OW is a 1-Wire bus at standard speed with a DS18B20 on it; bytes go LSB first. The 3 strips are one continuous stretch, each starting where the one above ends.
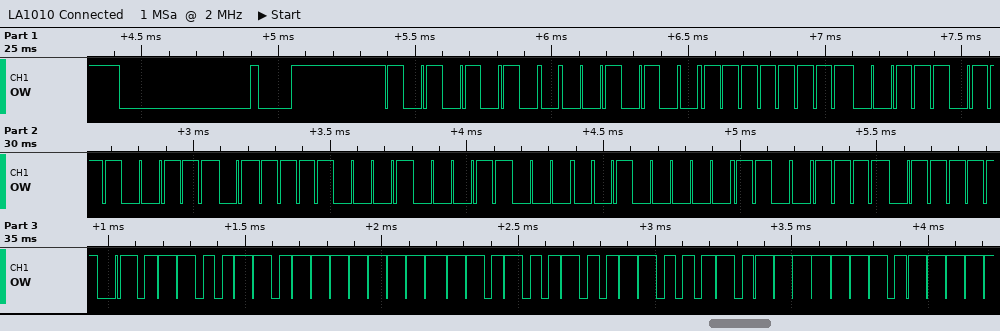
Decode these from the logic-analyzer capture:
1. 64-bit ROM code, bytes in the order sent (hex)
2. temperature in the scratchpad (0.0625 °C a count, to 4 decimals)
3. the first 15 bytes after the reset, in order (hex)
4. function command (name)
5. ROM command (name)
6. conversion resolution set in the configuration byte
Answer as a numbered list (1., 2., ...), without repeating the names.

1. 28 FF DC B9 8F 18 04 F3
2. -9.6250 °C
3. 55 28 FF DC B9 8F 18 04 F3 BE 66 FF 4B 46 7F
4. Read Scratchpad
5. Match ROM
6. 12 bits
